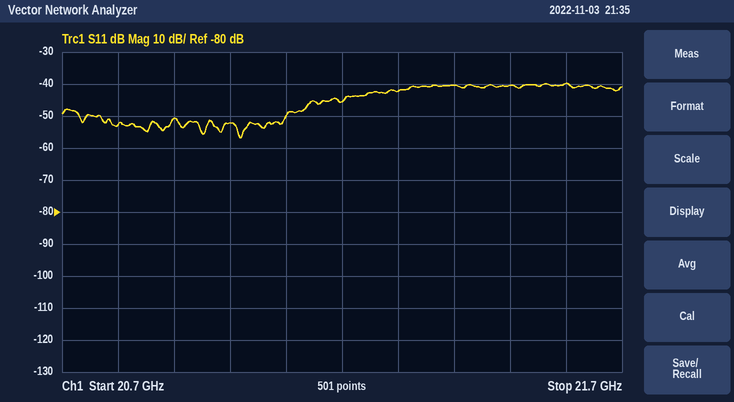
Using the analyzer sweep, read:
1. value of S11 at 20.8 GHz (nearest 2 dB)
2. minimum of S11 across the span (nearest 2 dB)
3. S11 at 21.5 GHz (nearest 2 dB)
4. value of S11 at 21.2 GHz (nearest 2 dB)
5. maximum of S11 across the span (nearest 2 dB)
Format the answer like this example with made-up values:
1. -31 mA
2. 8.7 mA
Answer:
1. -52 dB
2. -56 dB
3. -40 dB
4. -46 dB
5. -40 dB
